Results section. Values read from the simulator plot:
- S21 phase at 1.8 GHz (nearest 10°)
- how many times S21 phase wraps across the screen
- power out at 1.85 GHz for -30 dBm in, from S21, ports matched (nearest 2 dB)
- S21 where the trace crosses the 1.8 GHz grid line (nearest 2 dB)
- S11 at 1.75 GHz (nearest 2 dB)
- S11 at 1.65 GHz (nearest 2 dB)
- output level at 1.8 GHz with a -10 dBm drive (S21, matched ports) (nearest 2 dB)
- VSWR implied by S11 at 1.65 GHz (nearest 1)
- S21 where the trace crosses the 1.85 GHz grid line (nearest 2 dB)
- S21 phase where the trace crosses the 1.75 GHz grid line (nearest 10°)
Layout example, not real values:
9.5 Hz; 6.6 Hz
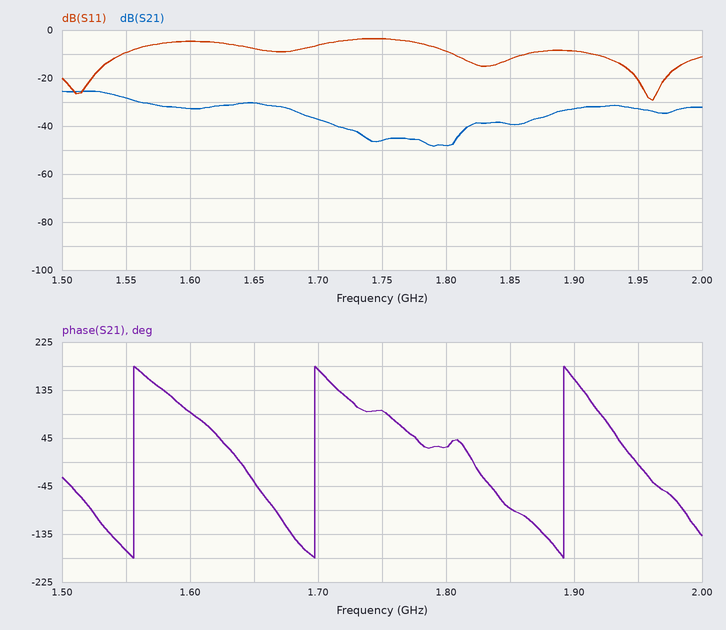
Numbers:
30°; 3; -70 dBm; -48 dB; -4 dB; -8 dB; -58 dBm; 2; -40 dB; 100°
